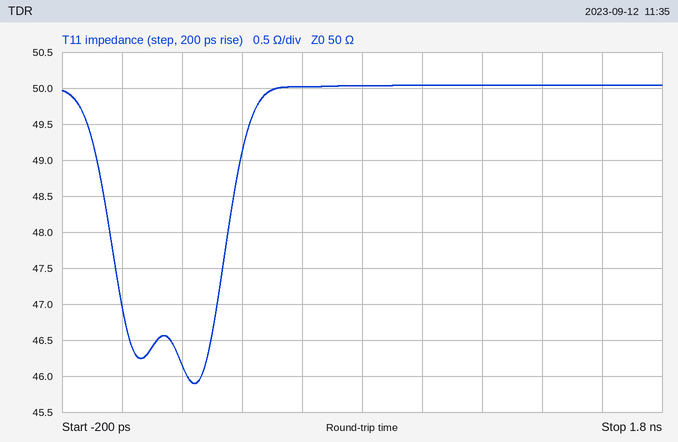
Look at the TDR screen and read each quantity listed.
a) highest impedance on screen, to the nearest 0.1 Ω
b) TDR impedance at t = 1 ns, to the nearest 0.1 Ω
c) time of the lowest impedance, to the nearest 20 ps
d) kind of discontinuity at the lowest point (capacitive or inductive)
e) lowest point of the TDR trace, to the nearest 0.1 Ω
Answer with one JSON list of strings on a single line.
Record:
["50.0 Ω", "50.0 Ω", "240 ps", "capacitive", "45.9 Ω"]
